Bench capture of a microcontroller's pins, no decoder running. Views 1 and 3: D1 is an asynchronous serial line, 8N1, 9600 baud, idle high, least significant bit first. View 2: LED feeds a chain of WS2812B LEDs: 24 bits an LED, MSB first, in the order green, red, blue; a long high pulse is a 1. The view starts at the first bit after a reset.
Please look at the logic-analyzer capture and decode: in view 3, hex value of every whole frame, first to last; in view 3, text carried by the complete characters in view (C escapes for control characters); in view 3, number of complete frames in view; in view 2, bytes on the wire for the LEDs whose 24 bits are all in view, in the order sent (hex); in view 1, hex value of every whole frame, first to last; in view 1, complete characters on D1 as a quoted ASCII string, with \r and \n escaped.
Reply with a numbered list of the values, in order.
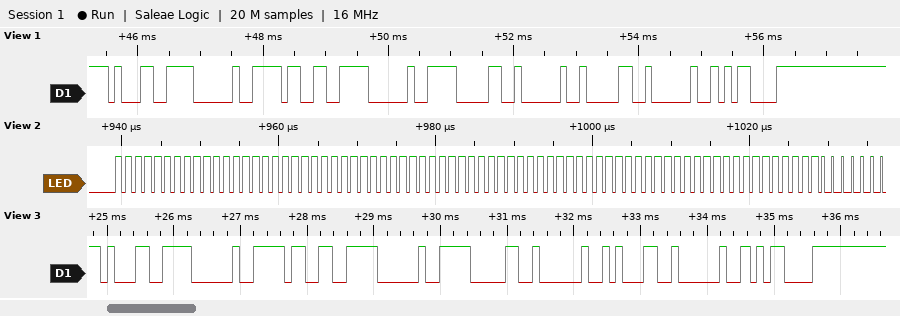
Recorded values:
1. 31 20 33 20 30 20 31 20 0D
2. "1 3 0 1 \r"
3. 9
4. FF FF FF FF FF FF FF FF FF
5. 31 20 33 20 30 20 30 20 0D
6. "1 3 0 0 \r"
